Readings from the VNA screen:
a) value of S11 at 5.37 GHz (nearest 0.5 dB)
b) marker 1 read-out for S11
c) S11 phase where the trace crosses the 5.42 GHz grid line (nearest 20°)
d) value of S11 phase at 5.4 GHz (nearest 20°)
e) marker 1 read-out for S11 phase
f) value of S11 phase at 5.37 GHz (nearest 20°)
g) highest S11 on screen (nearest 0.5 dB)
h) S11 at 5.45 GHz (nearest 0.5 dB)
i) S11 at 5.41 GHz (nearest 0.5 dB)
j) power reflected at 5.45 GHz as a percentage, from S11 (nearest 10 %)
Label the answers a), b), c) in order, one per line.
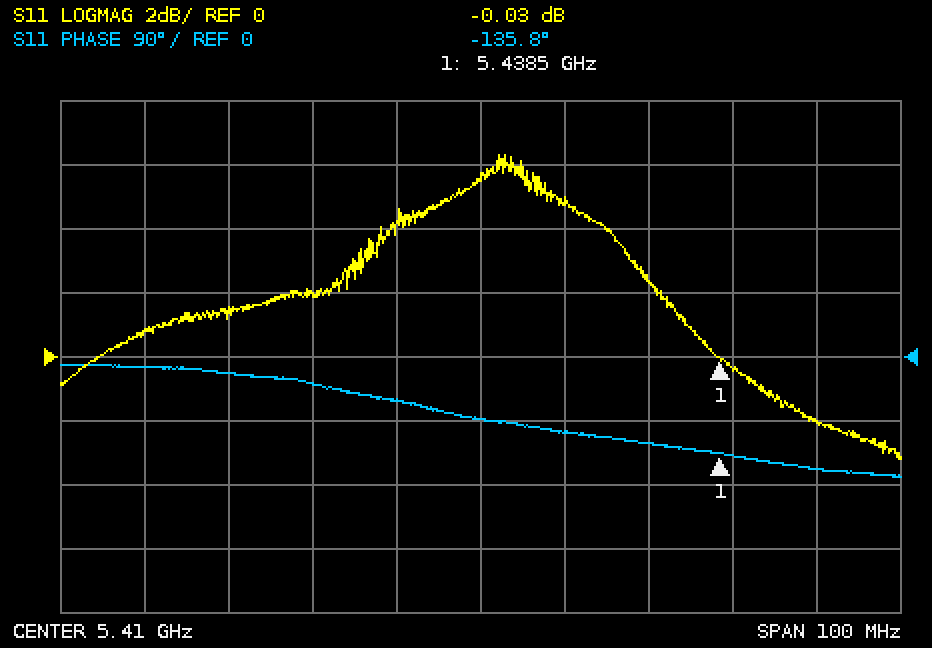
a) 1.0 dB
b) -0.03 dB
c) -100°
d) -60°
e) -135.8°
f) -20°
g) 6.5 dB
h) -2.0 dB
i) 5.5 dB
j) 60 %
